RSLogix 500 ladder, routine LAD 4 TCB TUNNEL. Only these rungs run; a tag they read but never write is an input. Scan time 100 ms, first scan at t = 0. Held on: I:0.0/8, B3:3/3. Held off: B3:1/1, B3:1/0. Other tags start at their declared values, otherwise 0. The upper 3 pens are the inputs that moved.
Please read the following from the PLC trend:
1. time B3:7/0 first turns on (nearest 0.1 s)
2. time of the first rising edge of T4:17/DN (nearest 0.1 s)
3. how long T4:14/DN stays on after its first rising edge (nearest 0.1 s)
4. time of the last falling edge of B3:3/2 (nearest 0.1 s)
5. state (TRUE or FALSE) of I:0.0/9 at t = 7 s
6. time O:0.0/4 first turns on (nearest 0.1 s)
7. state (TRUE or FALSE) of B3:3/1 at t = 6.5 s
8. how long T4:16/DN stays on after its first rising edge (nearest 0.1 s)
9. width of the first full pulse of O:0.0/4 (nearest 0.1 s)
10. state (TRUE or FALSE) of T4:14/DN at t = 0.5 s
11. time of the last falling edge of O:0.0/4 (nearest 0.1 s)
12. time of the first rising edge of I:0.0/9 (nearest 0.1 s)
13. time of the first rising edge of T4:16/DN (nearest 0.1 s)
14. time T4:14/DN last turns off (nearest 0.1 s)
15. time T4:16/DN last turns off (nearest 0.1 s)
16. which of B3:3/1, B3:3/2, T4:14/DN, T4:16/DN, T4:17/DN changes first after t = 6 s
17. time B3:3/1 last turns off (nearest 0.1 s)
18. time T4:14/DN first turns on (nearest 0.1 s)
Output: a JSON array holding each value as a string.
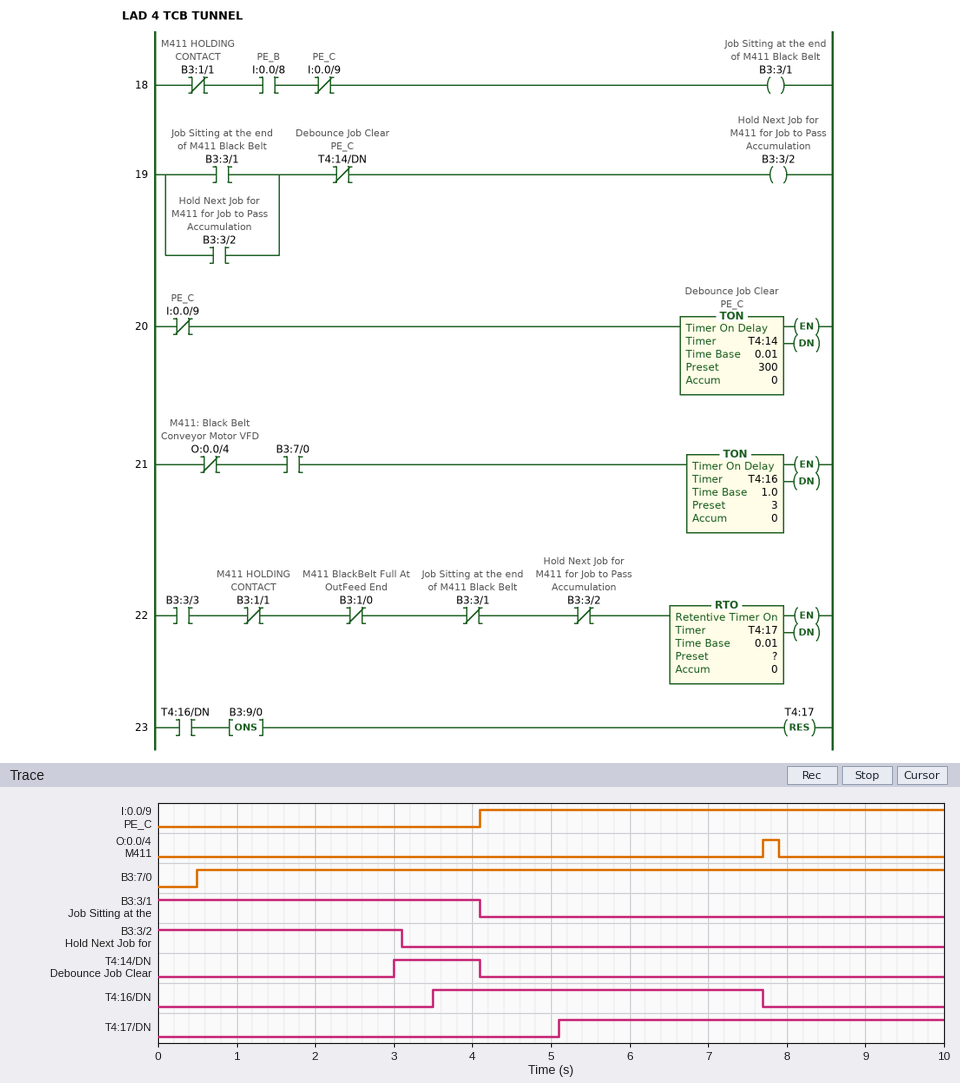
["0.5 s", "5.1 s", "1.1 s", "3.1 s", "TRUE", "7.7 s", "FALSE", "4.2 s", "0.2 s", "FALSE", "7.9 s", "4.1 s", "3.5 s", "4.1 s", "7.7 s", "T4:16/DN", "4.1 s", "3.0 s"]
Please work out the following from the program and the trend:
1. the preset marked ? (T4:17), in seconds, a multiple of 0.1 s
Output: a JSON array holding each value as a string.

["1.0 s"]
